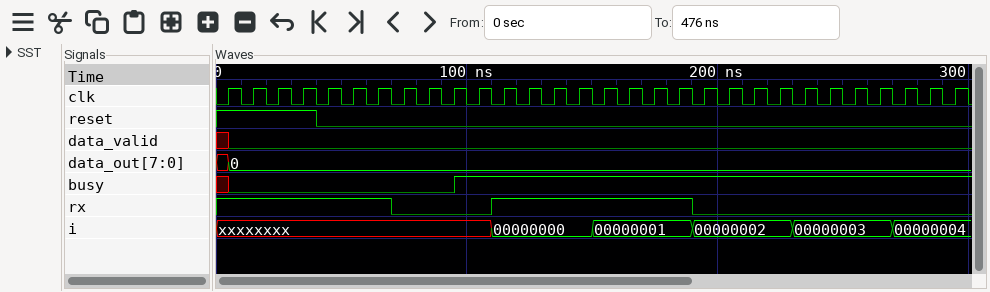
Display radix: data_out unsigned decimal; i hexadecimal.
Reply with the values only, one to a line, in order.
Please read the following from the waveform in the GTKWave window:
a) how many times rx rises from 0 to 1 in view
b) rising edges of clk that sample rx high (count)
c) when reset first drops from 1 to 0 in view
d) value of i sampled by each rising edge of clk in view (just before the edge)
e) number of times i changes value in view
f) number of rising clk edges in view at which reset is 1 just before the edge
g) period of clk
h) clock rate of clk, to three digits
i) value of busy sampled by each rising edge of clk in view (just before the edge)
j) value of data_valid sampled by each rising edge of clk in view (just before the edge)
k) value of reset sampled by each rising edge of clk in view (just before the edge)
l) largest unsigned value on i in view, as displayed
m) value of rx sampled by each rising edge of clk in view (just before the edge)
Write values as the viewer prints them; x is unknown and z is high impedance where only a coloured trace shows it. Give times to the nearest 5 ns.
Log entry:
1
15
40 ns
xxxxxxxx, xxxxxxxx, xxxxxxxx, xxxxxxxx, xxxxxxxx, xxxxxxxx, xxxxxxxx, xxxxxxxx, xxxxxxxx, xxxxxxxx, xxxxxxxx, 00000000, 00000000, 00000000, 00000000, 00000001, 00000001, 00000001, 00000001, 00000002, 00000002, 00000002, 00000002, 00000003, 00000003, 00000003, 00000003, 00000004, 00000004, 00000004
5
4
10 ns
100 MHz
x 0 0 0 0 0 0 0 0 0 1 1 1 1 1 1 1 1 1 1 1 1 1 1 1 1 1 1 1 1
x 0 0 0 0 0 0 0 0 0 0 0 0 0 0 0 0 0 0 0 0 0 0 0 0 0 0 0 0 0
1 1 1 1 0 0 0 0 0 0 0 0 0 0 0 0 0 0 0 0 0 0 0 0 0 0 0 0 0 0
00000004
1 1 1 1 1 1 1 0 0 0 0 1 1 1 1 1 1 1 1 0 0 0 0 0 0 0 0 0 0 0
